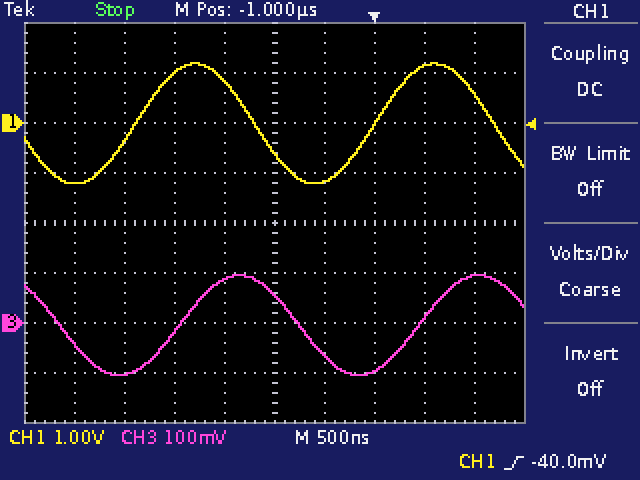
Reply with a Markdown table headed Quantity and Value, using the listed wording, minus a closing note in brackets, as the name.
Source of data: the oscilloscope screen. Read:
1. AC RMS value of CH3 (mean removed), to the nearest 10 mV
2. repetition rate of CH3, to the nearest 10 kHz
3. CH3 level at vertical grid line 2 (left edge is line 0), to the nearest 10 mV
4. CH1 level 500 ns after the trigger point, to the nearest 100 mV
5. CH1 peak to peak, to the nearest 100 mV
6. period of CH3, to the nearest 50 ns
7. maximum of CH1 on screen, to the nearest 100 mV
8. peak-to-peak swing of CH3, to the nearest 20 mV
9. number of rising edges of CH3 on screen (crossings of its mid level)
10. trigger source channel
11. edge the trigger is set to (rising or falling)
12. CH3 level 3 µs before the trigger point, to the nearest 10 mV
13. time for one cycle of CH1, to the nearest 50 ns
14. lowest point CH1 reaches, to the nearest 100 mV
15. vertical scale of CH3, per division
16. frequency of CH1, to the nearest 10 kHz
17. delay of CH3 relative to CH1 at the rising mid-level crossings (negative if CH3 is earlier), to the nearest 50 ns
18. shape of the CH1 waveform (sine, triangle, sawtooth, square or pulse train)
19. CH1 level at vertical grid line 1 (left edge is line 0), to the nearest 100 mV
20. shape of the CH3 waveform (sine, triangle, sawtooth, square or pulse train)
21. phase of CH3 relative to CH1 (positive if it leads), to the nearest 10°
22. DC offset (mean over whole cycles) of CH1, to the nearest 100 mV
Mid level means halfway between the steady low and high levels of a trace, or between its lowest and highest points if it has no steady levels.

| Quantity | Value |
|---|---|
| AC RMS value of CH3 (mean removed), to the nearest 10 mV | 70 mV |
| repetition rate of CH3, to the nearest 10 kHz | 420 kHz |
| CH3 level at vertical grid line 2 (left edge is line 0), to the nearest 10 mV | -100 mV |
| CH1 level 500 ns after the trigger point, to the nearest 100 mV | 1.1 V |
| CH1 peak to peak, to the nearest 100 mV | 2.4 V |
| period of CH3, to the nearest 50 ns | 2.40 µs |
| maximum of CH1 on screen, to the nearest 100 mV | 1.2 V |
| peak-to-peak swing of CH3, to the nearest 20 mV | 200 mV |
| number of rising edges of CH3 on screen | 2 |
| trigger source channel | CH1 |
| edge the trigger is set to | rising |
| CH3 level 3 µs before the trigger point, to the nearest 10 mV | -40 mV |
| time for one cycle of CH1, to the nearest 50 ns | 2.40 µs |
| lowest point CH1 reaches, to the nearest 100 mV | -1.2 V |
| vertical scale of CH3, per division | 100 mV |
| frequency of CH1, to the nearest 10 kHz | 420 kHz |
| delay of CH3 relative to CH1 at the rising mid-level crossings (negative if CH3 is earlier), to the nearest 50 ns | +450 ns |
| shape of the CH1 waveform | sine |
| CH1 level at vertical grid line 1 (left edge is line 0), to the nearest 100 mV | -1.2 V |
| shape of the CH3 waveform | sine |
| phase of CH3 relative to CH1 (positive if it leads), to the nearest 10° | -70° |
| DC offset (mean over whole cycles) of CH1, to the nearest 100 mV | 0.0 V |
